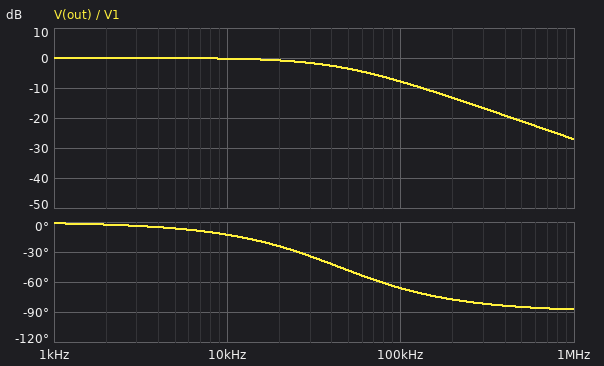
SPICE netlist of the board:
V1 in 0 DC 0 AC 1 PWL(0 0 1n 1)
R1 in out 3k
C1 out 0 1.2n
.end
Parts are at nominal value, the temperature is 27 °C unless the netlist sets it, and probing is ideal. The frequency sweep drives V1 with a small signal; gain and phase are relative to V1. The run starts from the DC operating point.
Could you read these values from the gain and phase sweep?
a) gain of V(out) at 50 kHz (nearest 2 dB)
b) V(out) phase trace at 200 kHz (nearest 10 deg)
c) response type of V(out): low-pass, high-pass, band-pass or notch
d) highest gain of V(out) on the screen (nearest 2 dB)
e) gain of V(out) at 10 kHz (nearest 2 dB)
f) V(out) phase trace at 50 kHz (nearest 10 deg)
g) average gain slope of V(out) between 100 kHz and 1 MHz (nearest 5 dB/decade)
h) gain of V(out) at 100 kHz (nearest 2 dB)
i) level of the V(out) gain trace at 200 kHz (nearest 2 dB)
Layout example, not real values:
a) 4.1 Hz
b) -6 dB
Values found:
a) -4 dB
b) -80 deg
c) low-pass
d) 0 dB
e) 0 dB
f) -50 deg
g) -20 dB/decade
h) -8 dB
i) -14 dB
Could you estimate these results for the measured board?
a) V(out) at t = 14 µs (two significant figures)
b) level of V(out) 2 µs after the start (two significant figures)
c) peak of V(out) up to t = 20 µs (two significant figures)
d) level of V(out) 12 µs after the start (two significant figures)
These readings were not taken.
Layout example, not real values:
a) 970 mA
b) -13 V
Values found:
a) 980 mV
b) 430 mV
c) 1.0 V
d) 960 mV
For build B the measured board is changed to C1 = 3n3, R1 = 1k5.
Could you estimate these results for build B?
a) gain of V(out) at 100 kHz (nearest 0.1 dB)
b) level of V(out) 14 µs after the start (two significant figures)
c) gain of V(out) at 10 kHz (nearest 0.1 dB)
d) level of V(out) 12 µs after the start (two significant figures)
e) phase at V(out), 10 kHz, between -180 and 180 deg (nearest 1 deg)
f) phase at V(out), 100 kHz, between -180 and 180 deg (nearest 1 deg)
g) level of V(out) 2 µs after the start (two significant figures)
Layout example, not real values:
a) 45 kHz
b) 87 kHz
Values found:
a) -10.3 dB
b) 940 mV
c) -0.4 dB
d) 910 mV
e) -17 deg
f) -72 deg
g) 330 mV
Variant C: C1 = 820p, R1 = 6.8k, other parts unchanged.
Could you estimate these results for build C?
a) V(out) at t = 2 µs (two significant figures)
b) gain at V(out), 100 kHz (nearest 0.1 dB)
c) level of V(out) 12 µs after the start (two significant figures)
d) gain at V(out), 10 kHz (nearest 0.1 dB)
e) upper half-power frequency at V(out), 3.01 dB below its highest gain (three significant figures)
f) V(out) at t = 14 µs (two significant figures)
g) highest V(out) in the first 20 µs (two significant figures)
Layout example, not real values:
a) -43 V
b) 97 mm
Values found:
a) 300 mV
b) -11.2 dB
c) 880 mV
d) -0.5 dB
e) 28.5 kHz
f) 920 mV
g) 970 mV
